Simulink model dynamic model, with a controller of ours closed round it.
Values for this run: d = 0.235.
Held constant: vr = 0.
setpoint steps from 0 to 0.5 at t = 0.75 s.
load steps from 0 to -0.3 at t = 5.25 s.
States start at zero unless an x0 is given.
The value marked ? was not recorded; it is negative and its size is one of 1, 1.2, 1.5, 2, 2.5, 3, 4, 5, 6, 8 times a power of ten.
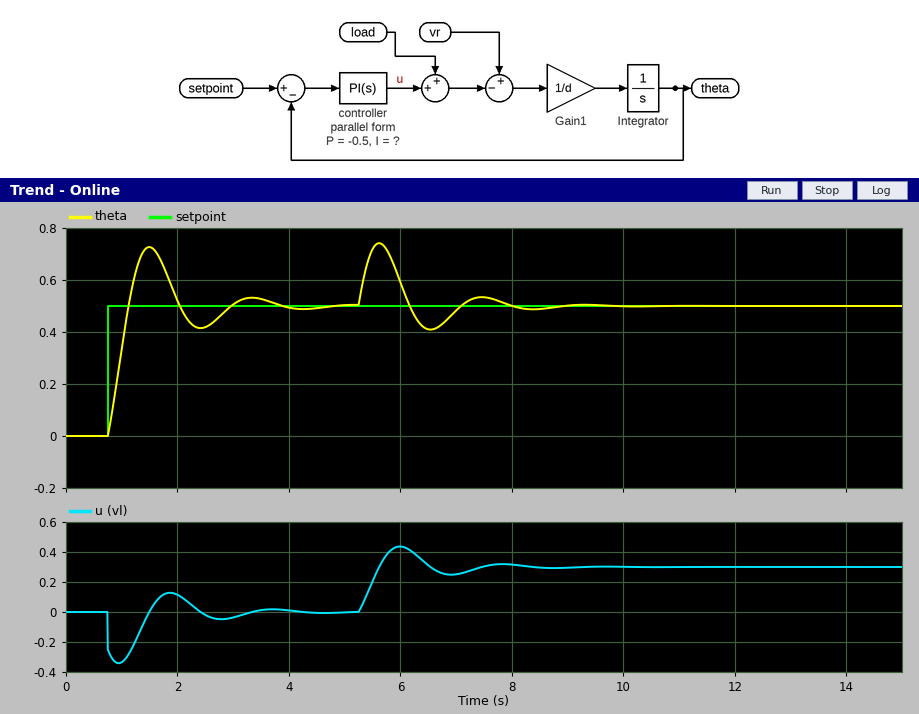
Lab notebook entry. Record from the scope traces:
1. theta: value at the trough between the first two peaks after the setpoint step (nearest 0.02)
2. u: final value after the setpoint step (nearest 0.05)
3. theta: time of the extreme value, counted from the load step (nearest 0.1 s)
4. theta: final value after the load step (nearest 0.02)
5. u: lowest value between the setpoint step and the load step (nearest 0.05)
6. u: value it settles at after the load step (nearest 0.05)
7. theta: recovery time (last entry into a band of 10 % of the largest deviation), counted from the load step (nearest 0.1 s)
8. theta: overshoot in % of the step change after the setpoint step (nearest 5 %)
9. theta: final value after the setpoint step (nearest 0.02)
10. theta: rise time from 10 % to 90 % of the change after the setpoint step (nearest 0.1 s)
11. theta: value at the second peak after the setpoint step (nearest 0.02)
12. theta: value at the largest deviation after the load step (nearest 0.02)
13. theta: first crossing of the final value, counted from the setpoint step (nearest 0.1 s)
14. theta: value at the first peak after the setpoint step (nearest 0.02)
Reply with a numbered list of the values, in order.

1. 0.42
2. 0.00
3. 0.4 s
4. 0.50
5. -0.35
6. 0.30
7. 2.5 s
8. 45 %
9. 0.50
10. 0.3 s
11. 0.54
12. 0.74
13. 0.4 s
14. 0.72
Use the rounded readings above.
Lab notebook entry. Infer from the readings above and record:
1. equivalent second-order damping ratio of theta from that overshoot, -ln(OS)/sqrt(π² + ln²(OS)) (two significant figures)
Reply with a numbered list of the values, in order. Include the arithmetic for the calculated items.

1. ln(0.45) = -0.799; 0.799 / sqrt(9.870 + 0.638) = 0.25
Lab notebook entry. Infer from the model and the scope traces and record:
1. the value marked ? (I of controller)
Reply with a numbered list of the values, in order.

1. -3
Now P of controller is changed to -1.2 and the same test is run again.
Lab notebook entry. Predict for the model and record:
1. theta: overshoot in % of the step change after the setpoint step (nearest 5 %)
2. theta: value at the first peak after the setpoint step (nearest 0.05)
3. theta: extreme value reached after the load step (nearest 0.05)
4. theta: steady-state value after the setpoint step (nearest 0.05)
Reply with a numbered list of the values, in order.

1. 20 %
2. 0.60
3. 0.65
4. 0.50
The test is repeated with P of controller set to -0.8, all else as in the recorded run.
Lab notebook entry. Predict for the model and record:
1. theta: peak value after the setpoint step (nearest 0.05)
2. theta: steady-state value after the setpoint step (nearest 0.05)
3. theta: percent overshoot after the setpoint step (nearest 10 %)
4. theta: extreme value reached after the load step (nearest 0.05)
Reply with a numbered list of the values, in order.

1. 0.65
2. 0.50
3. 30 %
4. 0.70
